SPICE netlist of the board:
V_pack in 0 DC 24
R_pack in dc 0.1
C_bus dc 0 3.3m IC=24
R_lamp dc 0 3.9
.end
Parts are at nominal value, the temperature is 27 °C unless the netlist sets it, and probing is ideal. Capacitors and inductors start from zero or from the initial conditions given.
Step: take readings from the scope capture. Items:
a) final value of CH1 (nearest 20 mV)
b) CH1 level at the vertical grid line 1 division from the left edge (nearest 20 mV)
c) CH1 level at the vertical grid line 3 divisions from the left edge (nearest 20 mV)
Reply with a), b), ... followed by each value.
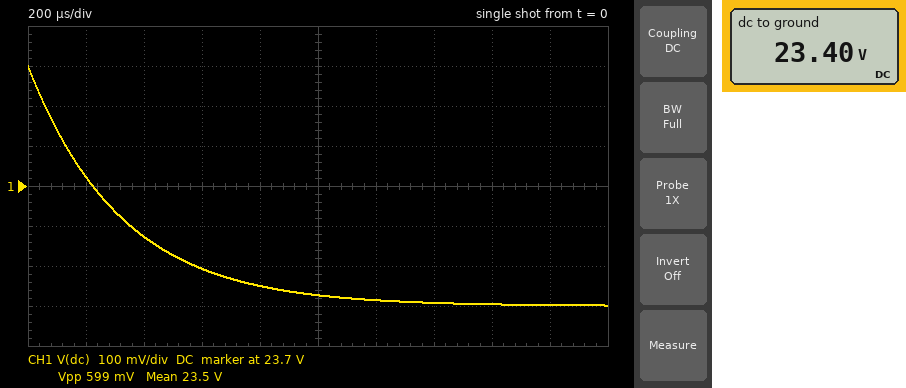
a) 23.40 V
b) 23.72 V
c) 23.50 V
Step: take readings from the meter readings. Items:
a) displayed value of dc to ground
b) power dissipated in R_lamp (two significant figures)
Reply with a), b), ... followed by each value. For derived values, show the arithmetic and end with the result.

a) 23.40 V
b) (23.4 V)^2 / 3.9 Ω = 140 W
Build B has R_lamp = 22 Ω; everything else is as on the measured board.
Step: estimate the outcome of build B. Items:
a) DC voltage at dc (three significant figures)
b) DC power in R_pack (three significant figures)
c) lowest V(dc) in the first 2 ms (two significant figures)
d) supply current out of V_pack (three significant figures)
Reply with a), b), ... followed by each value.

a) 23.9 V
b) 118 mW
c) 24 V
d) 1.09 A
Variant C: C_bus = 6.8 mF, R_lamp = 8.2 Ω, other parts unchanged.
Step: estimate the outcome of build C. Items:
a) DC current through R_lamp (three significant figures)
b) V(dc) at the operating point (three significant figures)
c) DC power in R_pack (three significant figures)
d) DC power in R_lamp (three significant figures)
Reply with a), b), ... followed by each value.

a) 2.89 A
b) 23.7 V
c) 836 mW
d) 68.6 W
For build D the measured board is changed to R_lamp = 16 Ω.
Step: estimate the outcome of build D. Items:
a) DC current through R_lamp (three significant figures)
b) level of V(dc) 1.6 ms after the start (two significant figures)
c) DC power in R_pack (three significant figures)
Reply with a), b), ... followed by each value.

a) 1.49 A
b) 24 V
c) 222 mW
